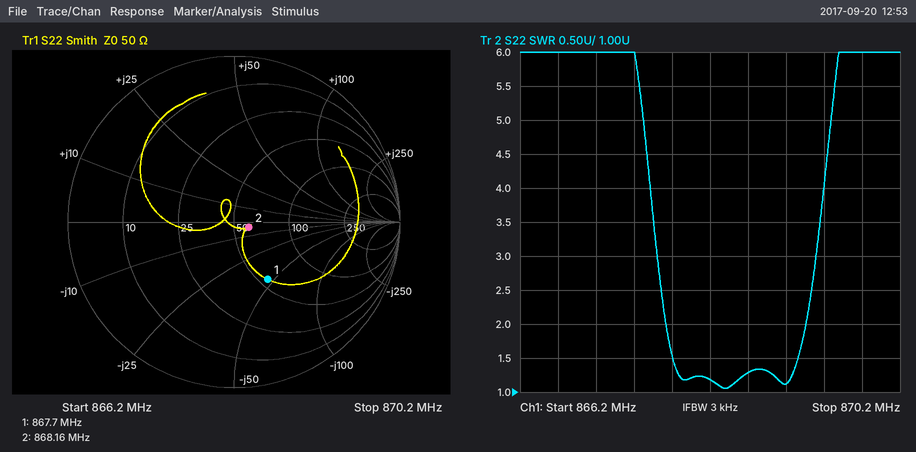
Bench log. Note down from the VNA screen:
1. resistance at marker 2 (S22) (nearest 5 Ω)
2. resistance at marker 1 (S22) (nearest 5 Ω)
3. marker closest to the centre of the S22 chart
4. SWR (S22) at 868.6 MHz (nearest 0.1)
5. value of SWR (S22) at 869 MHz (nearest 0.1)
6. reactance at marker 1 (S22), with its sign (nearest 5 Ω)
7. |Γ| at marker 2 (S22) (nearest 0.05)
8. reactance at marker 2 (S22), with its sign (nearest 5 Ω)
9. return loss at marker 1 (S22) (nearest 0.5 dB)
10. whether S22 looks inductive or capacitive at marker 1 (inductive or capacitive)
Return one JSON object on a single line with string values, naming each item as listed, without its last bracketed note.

{"resistance at marker 2 (S22)": "60 Ω", "resistance at marker 1 (S22)": "55 Ω", "marker closest to the centre of the S22 chart": "marker 2", "SWR (S22) at 868.6 MHz": "1.3", "value of SWR (S22) at 869 MHz": "1.1", "reactance at marker 1 (S22), with its sign": "-45 Ω", "|Γ| at marker 2 (S22)": "0.10", "reactance at marker 2 (S22), with its sign": "-5 Ω", "return loss at marker 1 (S22)": "8.0 dB", "whether S22 looks inductive or capacitive at marker 1": "capacitive"}
